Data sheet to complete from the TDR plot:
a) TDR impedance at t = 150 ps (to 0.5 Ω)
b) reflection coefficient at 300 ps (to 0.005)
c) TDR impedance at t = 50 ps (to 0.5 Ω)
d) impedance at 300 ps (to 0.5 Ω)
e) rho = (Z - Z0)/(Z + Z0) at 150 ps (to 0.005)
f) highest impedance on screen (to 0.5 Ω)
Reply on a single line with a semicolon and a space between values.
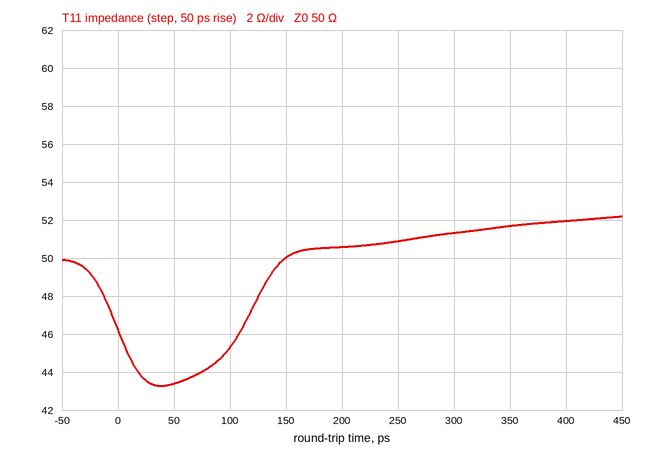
50.0 Ω; +0.015; 43.5 Ω; 51.5 Ω; 0.000; 52.0 Ω
